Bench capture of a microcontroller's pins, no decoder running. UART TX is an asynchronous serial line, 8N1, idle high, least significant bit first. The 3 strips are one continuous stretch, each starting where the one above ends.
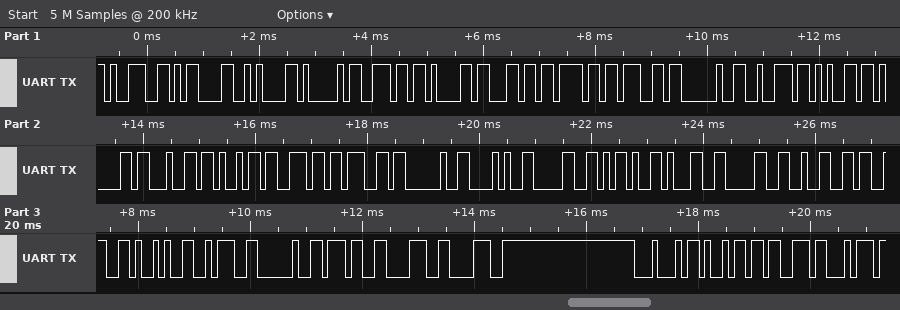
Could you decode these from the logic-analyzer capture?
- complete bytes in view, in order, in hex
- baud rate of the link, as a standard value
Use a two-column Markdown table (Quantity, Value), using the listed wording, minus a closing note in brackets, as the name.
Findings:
| Quantity | Value |
|---|---|
| complete bytes in view, in order, in hex | 0x39 0x0D 0x0A 0x41 0x6E 0x61 0x6C 0x6F 0x67 0x20 0x72 0x65 0x61 0x64 0x69 0x6E 0x67 0x20 0x28 0x30 0x2D 0x31 0x30 0x32 0x33 0x29 0x3A 0x20 0x37 0x38 0x38 0x44 0x69 0x73 0x74 |
| baud rate of the link, as a standard value | 9600 baud |
